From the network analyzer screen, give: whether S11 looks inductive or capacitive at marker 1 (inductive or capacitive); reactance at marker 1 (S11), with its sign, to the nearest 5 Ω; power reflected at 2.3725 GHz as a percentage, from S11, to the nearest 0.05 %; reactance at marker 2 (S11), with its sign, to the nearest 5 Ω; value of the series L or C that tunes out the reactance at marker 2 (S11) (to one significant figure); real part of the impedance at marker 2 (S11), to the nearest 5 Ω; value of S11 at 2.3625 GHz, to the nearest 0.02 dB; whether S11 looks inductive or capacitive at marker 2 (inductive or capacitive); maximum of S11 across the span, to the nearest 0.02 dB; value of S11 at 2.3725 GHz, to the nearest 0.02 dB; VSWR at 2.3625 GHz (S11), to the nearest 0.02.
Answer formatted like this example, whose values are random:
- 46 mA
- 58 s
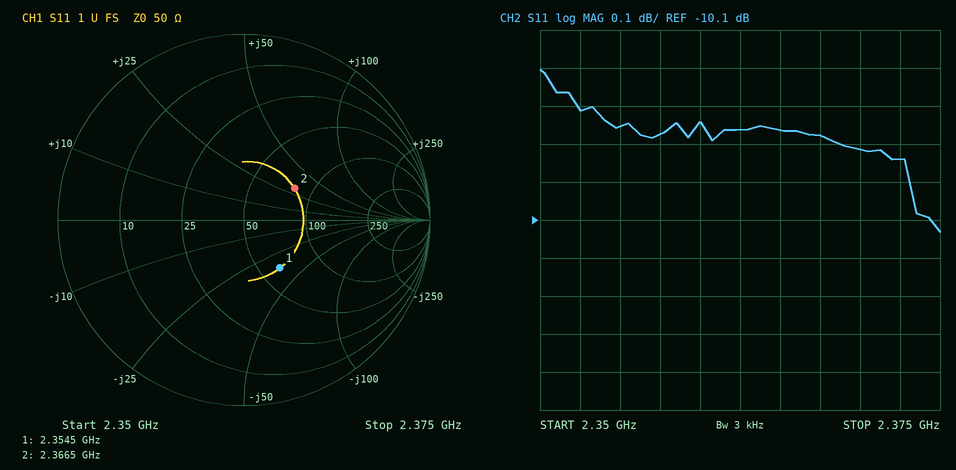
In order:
- capacitive
- -35 Ω
- 10.15 %
- +30 Ω
- 2 pF
- 80 Ω
- -9.86 dB
- inductive
- -9.70 dB
- -9.94 dB
- 1.94
